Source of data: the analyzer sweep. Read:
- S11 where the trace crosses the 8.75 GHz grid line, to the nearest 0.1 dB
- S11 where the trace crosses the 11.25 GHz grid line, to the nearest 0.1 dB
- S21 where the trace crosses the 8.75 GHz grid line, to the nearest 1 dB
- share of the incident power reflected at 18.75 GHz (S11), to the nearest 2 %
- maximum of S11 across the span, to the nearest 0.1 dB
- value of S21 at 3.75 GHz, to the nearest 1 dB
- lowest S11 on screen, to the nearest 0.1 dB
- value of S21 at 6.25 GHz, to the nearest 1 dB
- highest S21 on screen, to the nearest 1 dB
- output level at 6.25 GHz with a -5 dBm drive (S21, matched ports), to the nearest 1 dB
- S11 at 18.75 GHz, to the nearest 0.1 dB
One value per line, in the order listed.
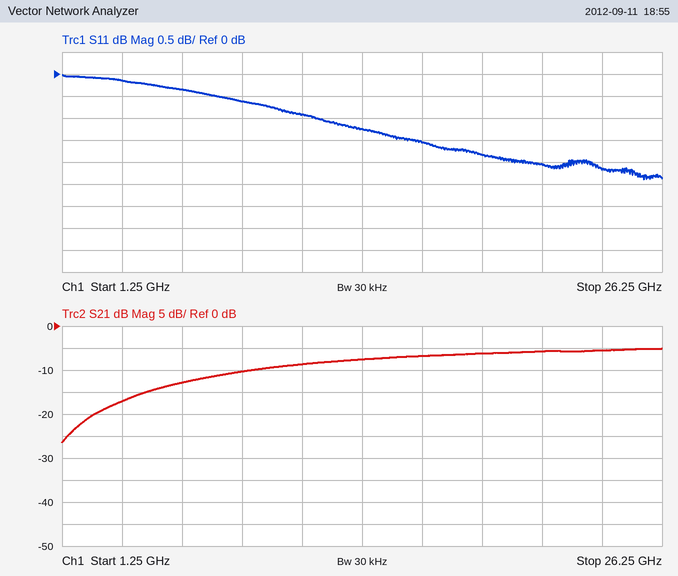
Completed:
-0.6 dB
-0.9 dB
-10 dB
66 %
0.0 dB
-17 dB
-2.4 dB
-13 dB
-5 dB
-18 dBm
-1.8 dB
